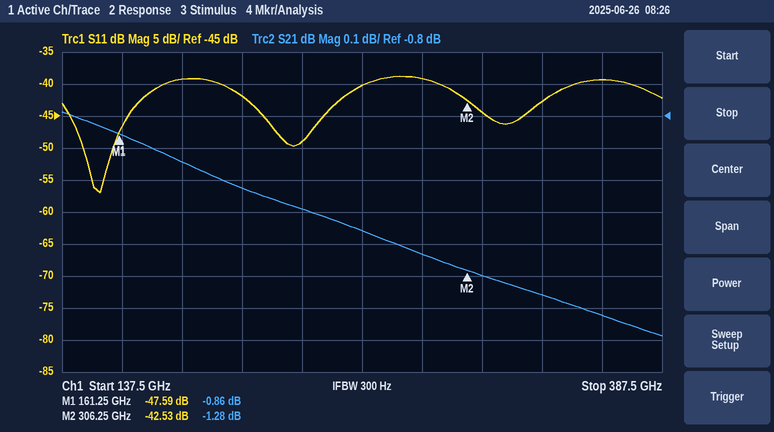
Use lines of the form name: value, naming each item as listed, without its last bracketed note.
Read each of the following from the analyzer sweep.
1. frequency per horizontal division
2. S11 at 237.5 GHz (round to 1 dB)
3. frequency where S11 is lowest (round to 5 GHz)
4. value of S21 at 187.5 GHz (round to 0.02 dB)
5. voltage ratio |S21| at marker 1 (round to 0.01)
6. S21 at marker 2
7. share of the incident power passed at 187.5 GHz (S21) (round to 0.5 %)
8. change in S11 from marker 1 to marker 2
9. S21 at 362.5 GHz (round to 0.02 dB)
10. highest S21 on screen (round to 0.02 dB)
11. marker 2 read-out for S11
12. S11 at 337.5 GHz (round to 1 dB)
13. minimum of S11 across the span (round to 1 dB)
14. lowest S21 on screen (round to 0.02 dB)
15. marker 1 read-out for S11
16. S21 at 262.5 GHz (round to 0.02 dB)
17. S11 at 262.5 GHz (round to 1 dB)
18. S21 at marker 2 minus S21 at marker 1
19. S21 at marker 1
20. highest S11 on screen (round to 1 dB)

frequency per horizontal division: 25 GHz
S11 at 237.5 GHz: -49 dB
frequency where S11 is lowest: 155 GHz
value of S21 at 187.5 GHz: -0.94 dB
voltage ratio |S21| at marker 1: 0.91
S21 at marker 2: -1.28 dB
share of the incident power passed at 187.5 GHz (S21): 80.5 %
change in S11 from marker 1 to marker 2: 5.06 dB
S21 at 362.5 GHz: -1.42 dB
highest S21 on screen: -0.78 dB
marker 2 read-out for S11: -42.53 dB
S11 at 337.5 GHz: -43 dB
minimum of S11 across the span: -57 dB
lowest S21 on screen: -1.48 dB
marker 1 read-out for S11: -47.59 dB
S21 at 262.5 GHz: -1.16 dB
S11 at 262.5 GHz: -40 dB
S21 at marker 2 minus S21 at marker 1: -0.42 dB
S21 at marker 1: -0.86 dB
highest S11 on screen: -39 dB
